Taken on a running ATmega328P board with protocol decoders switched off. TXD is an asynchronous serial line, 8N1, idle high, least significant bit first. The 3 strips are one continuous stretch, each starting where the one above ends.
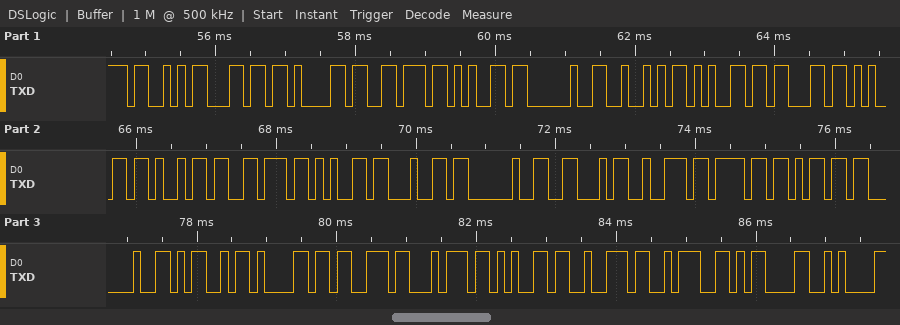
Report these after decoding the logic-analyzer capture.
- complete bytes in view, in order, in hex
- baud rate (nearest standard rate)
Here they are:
53 6C 61 76 65 20 52 65 63 65 69 76 65 64 20 46 72 6F 6D 20 4D 61 73 74 65 72 3A 0D 0A
9600 baud
